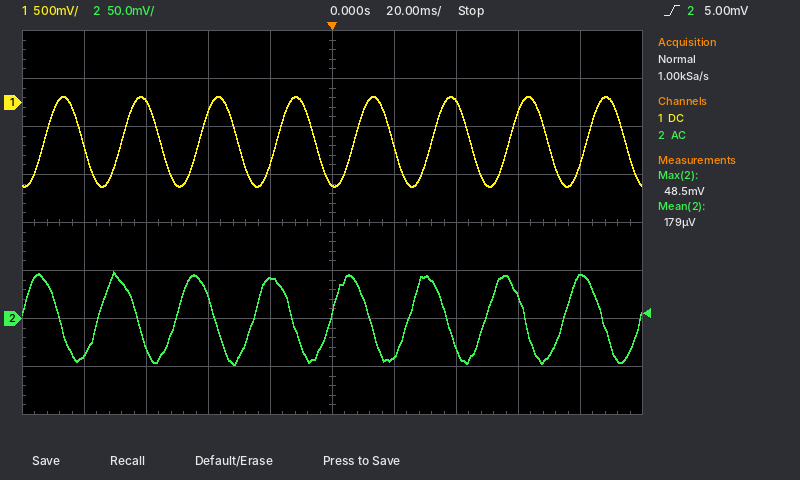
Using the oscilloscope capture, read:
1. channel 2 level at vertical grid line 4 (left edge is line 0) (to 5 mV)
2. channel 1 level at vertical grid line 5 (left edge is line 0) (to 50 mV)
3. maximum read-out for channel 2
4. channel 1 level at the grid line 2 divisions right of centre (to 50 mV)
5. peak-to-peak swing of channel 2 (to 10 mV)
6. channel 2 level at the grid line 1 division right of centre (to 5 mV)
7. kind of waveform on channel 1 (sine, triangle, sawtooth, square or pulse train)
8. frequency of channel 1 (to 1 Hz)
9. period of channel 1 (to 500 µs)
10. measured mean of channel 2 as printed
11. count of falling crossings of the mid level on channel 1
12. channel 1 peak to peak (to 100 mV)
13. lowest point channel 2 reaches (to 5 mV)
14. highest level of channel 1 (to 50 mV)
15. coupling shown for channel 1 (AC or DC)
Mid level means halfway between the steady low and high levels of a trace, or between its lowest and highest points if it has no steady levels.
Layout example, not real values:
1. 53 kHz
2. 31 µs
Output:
1. 40 mV
2. -850 mV
3. 48.5 mV
4. 0 mV
5. 100 mV
6. -40 mV
7. sine
8. 40 Hz
9. 25.0 ms
10. 179 µV
11. 8
12. 900 mV
13. -50 mV
14. 50 mV
15. DC
